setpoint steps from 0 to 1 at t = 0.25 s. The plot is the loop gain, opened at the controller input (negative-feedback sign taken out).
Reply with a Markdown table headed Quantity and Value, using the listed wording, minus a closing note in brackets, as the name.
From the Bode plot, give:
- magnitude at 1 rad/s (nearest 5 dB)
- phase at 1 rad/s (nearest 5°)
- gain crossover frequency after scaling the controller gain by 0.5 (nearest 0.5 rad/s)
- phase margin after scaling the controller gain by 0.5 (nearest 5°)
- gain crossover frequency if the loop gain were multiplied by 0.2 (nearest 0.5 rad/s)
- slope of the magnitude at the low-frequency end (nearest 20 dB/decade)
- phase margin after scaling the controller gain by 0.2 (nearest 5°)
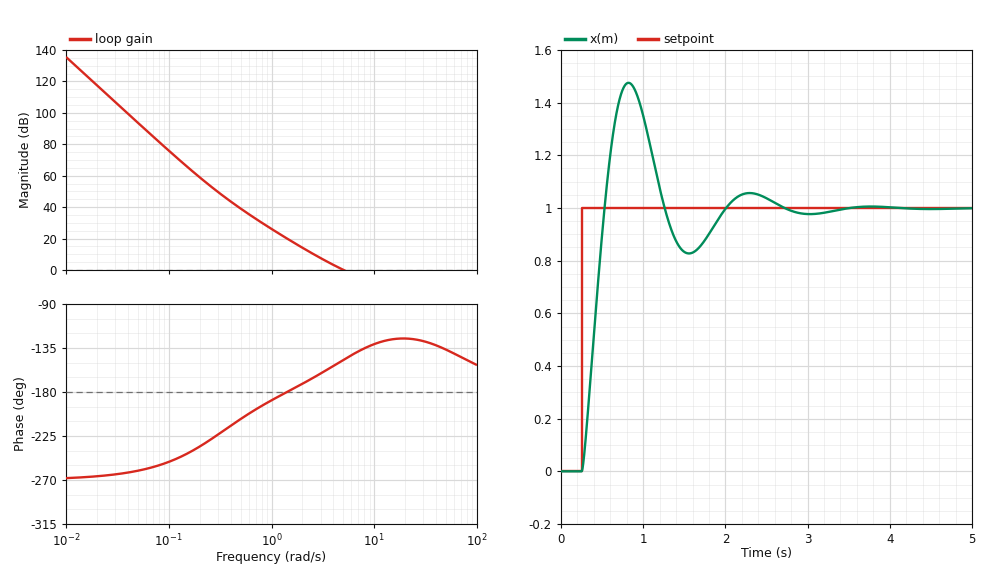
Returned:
| Quantity | Value |
|---|---|
| magnitude at 1 rad/s | 25 dB |
| phase at 1 rad/s | -190° |
| gain crossover frequency after scaling the controller gain by 0.5 | 3.5 rad/s |
| phase margin after scaling the controller gain by 0.5 | 20° |
| gain crossover frequency if the loop gain were multiplied by 0.2 | 2.0 rad/s |
| slope of the magnitude at the low-frequency end | -60 dB/decade |
| phase margin after scaling the controller gain by 0.2 | 10° |
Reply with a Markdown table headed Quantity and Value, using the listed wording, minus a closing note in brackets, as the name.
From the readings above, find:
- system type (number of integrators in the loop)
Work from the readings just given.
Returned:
| Quantity | Value |
|---|---|
| system type | 3 |
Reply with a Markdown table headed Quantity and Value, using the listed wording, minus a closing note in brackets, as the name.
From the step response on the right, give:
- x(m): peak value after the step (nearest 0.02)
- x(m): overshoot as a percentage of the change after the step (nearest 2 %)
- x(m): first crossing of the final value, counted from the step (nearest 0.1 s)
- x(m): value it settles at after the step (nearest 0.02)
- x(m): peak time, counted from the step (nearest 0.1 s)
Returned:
| Quantity | Value |
|---|---|
| x(m): peak value after the step | 1.48 |
| x(m): overshoot as a percentage of the change after the step | 48 % |
| x(m): first crossing of the final value, counted from the step | 0.3 s |
| x(m): value it settles at after the step | 1.00 |
| x(m): peak time, counted from the step | 0.6 s |
